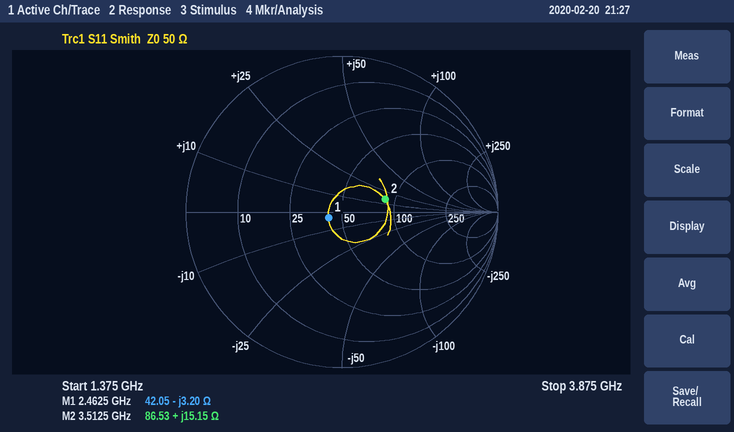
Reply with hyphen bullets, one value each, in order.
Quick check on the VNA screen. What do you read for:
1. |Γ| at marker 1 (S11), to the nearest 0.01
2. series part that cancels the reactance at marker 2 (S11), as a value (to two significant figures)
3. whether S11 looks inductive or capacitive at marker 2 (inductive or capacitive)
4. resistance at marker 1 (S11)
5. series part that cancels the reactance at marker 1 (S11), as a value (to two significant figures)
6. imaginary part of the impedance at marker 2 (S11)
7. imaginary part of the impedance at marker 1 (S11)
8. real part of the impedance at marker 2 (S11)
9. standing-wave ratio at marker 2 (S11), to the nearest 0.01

- 0.09
- 3.0 pF
- inductive
- 42.05 Ω
- 210 pH
- +15.15 Ω
- -3.20 Ω
- 86.53 Ω
- 1.81
